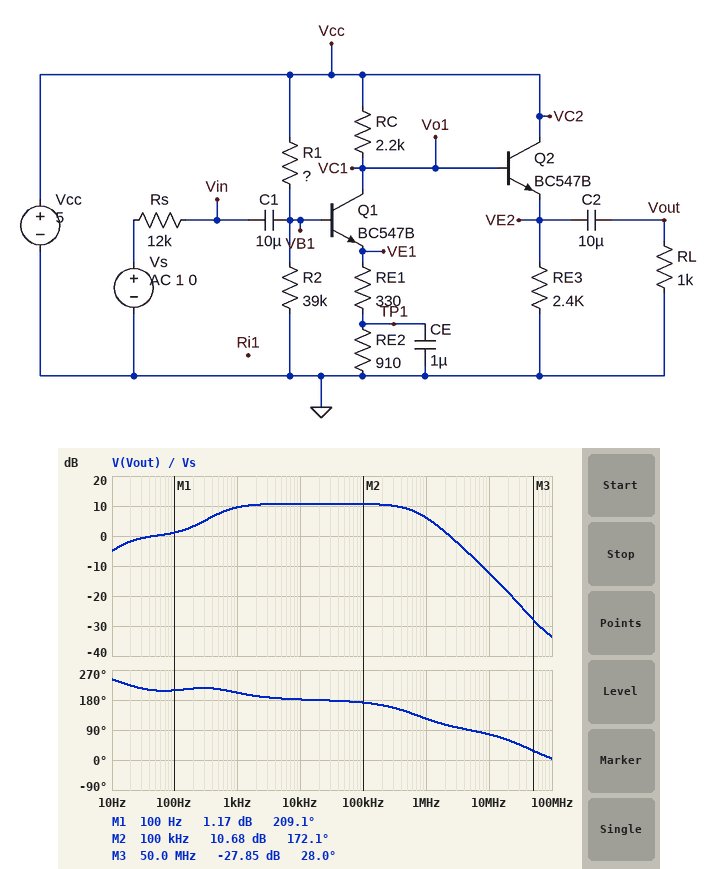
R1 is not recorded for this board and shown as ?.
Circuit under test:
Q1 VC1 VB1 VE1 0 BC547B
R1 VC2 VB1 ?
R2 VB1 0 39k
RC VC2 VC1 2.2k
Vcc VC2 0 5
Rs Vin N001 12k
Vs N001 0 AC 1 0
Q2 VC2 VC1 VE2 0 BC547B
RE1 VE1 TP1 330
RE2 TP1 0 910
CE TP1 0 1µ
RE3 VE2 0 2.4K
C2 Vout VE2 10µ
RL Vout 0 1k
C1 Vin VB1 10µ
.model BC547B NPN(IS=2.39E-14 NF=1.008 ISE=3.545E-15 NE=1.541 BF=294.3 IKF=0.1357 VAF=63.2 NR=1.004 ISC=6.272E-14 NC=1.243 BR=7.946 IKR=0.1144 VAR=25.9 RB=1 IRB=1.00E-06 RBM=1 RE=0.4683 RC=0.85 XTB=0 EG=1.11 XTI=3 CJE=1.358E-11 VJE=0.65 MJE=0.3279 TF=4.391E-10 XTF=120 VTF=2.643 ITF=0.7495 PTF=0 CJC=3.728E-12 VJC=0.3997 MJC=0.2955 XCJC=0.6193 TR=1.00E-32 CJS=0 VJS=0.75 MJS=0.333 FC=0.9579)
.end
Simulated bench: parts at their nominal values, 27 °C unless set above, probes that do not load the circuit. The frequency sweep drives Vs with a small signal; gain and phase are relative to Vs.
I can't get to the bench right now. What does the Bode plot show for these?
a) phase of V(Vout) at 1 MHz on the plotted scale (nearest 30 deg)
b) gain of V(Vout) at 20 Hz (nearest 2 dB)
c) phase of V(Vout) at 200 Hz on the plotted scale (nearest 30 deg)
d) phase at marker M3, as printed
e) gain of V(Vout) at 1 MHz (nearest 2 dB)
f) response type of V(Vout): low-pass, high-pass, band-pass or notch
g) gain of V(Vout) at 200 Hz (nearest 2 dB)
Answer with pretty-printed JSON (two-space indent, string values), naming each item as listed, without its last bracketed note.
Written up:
{
  "phase of V(Vout) at 1 MHz on the plotted scale": "120 deg",
  "gain of V(Vout) at 20 Hz": "-2 dB",
  "phase of V(Vout) at 200 Hz on the plotted scale": "210 deg",
  "phase at marker M3, as printed": "28.0 deg",
  "gain of V(Vout) at 1 MHz": "6 dB",
  "response type of V(Vout): low-pass, high-pass, band-pass or notch": "band-pass",
  "gain of V(Vout) at 200 Hz": "4 dB"
}
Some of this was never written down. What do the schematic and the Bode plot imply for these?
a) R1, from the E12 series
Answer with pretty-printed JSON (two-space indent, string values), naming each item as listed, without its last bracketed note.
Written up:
{
  "R1, from the E12 series": "47 kΩ"
}
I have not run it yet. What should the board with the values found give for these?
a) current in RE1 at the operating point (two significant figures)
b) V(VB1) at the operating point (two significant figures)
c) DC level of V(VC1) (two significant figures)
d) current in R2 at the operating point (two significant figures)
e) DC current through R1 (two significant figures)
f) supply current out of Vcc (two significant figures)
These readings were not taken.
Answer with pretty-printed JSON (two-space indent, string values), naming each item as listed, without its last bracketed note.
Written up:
{
  "current in RE1 at the operating point": "1.2 mA",
  "V(VB1) at the operating point": "2.2 V",
  "DC level of V(VC1)": "2.3 V",
  "current in R2 at the operating point": "56 µA",
  "DC current through R1": "60 µA",
  "supply current out of Vcc": "2.0 mA"
}
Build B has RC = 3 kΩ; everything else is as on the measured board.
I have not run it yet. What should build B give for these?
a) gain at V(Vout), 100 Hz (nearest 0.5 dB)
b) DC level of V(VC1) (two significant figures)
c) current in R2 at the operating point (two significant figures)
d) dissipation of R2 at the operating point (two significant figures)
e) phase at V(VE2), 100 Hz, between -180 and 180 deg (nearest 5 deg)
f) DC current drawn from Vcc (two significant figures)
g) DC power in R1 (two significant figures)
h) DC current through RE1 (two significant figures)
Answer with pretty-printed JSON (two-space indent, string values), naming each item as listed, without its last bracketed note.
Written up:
{
  "gain at V(Vout), 100 Hz": "-14.0 dB",
  "DC level of V(VC1)": "1.5 V",
  "current in R2 at the operating point": "53 µA",
  "dissipation of R2 at the operating point": "110 µW",
  "phase at V(VE2), 100 Hz, between -180 and 180 deg": "-165 deg",
  "DC current drawn from Vcc": "1.6 mA",
  "DC power in R1": "180 µW",
  "DC current through RE1": "1.2 mA"
}
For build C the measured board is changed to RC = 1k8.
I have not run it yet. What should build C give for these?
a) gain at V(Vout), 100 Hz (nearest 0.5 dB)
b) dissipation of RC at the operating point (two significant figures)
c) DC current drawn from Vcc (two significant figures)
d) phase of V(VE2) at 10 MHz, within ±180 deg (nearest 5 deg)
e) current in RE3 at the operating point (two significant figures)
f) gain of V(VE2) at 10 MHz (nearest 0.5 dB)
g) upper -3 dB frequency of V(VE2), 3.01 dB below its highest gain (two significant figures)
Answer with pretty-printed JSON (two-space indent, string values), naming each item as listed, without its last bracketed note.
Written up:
{
  "gain at V(Vout), 100 Hz": "-0.5 dB",
  "dissipation of RC at the operating point": "2.7 mW",
  "DC current drawn from Vcc": "2.2 mA",
  "phase of V(VE2) at 10 MHz, within ±180 deg": "80 deg",
  "current in RE3 at the operating point": "890 µA",
  "gain of V(VE2) at 10 MHz": "-11.5 dB",
  "upper -3 dB frequency of V(VE2), 3.01 dB below its highest gain": "980 kHz"
}
